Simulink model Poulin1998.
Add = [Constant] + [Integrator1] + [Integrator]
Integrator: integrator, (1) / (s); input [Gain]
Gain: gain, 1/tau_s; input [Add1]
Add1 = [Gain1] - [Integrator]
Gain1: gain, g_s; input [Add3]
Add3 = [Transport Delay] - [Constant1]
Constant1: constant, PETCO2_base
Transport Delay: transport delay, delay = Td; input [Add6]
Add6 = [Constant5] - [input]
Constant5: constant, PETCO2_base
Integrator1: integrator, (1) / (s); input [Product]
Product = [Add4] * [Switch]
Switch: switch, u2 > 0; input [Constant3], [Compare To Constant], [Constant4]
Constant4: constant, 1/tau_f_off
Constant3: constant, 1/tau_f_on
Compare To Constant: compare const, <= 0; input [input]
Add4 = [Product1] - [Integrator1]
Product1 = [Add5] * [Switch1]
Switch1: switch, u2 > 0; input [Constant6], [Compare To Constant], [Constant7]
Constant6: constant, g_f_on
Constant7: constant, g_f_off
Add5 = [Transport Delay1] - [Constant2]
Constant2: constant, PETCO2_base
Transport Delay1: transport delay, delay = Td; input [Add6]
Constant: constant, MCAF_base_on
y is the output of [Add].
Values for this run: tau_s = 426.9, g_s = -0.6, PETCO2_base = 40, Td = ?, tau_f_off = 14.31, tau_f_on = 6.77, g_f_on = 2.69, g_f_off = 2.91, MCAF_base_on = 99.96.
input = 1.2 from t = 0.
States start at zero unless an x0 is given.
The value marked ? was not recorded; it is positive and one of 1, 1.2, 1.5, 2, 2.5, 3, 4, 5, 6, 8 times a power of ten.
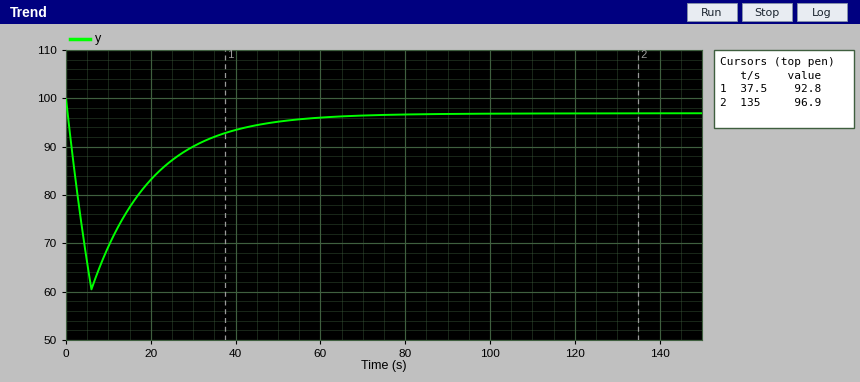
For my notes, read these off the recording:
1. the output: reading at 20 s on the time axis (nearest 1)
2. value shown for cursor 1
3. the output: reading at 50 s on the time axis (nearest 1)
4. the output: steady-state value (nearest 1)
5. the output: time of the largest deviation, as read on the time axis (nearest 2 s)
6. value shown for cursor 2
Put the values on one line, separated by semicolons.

83; 92.8; 95; 97; 6 s; 96.9
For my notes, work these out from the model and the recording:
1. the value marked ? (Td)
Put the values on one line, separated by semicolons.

6
